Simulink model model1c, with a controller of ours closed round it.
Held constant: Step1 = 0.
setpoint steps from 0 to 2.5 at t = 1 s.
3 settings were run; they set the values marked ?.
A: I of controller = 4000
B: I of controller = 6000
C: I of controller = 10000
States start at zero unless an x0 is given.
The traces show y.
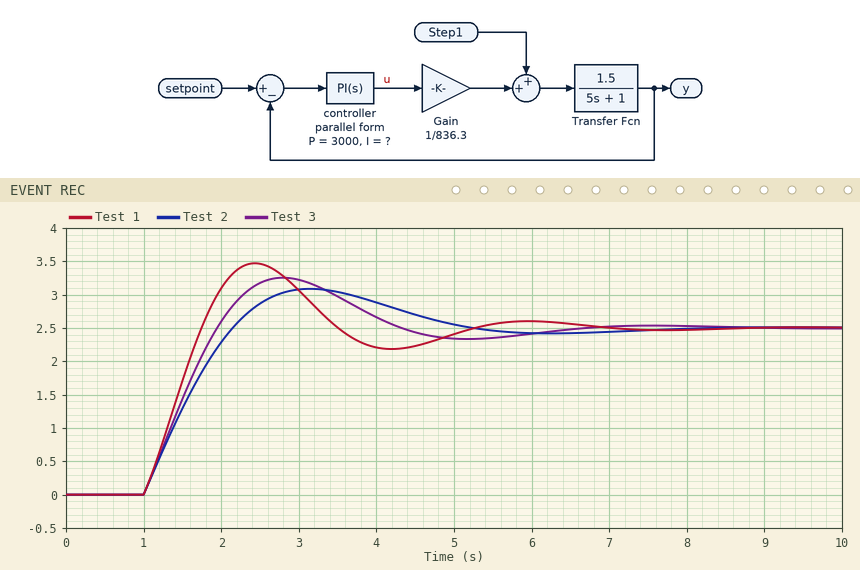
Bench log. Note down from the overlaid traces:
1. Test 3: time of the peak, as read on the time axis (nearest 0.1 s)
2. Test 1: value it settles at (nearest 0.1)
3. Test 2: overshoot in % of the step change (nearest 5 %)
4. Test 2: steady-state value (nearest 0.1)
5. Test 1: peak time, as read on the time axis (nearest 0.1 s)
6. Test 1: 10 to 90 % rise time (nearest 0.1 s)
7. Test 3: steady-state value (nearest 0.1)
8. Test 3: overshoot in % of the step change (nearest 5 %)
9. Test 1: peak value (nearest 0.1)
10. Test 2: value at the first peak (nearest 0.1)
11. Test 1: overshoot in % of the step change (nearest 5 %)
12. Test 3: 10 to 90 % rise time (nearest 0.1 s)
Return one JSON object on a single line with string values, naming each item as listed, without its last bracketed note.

{"Test 3: time of the peak, as read on the time axis": "2.8 s", "Test 1: value it settles at": "2.5", "Test 2: overshoot in % of the step change": "25 %", "Test 2: steady-state value": "2.5", "Test 1: peak time, as read on the time axis": "2.4 s", "Test 1: 10 to 90 % rise time": "0.6 s", "Test 3: steady-state value": "2.5", "Test 3: overshoot in % of the step change": "30 %", "Test 1: peak value": "3.5", "Test 2: value at the first peak": "3.1", "Test 1: overshoot in % of the step change": "40 %", "Test 3: 10 to 90 % rise time": "0.7 s"}
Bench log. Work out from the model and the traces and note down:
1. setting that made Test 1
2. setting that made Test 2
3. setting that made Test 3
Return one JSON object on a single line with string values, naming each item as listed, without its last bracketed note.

{"setting that made Test 1": "C", "setting that made Test 2": "A", "setting that made Test 3": "B"}
